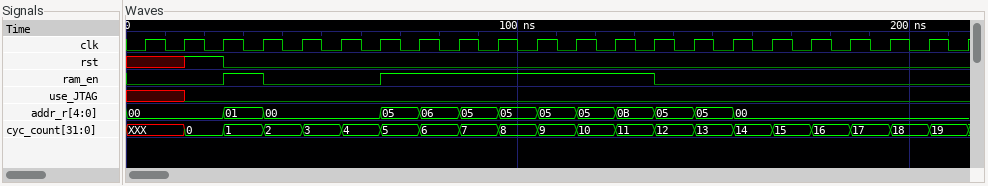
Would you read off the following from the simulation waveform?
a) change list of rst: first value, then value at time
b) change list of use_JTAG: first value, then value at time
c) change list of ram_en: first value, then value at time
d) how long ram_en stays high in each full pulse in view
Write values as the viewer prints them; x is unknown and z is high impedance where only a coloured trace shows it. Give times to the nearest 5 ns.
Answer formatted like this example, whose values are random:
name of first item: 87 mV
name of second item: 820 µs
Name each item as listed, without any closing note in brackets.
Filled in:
change list of rst: first value, then value at time: x, 1 at 15 ns, 0 at 25 ns
change list of use_JTAG: first value, then value at time: x, 0 at 15 ns
change list of ram_en: first value, then value at time: 0, 1 at 25 ns, 0 at 35 ns, 1 at 65 ns, 0 at 135 ns
how long ram_en stays high in each full pulse in view: 10 ns, 70 ns
